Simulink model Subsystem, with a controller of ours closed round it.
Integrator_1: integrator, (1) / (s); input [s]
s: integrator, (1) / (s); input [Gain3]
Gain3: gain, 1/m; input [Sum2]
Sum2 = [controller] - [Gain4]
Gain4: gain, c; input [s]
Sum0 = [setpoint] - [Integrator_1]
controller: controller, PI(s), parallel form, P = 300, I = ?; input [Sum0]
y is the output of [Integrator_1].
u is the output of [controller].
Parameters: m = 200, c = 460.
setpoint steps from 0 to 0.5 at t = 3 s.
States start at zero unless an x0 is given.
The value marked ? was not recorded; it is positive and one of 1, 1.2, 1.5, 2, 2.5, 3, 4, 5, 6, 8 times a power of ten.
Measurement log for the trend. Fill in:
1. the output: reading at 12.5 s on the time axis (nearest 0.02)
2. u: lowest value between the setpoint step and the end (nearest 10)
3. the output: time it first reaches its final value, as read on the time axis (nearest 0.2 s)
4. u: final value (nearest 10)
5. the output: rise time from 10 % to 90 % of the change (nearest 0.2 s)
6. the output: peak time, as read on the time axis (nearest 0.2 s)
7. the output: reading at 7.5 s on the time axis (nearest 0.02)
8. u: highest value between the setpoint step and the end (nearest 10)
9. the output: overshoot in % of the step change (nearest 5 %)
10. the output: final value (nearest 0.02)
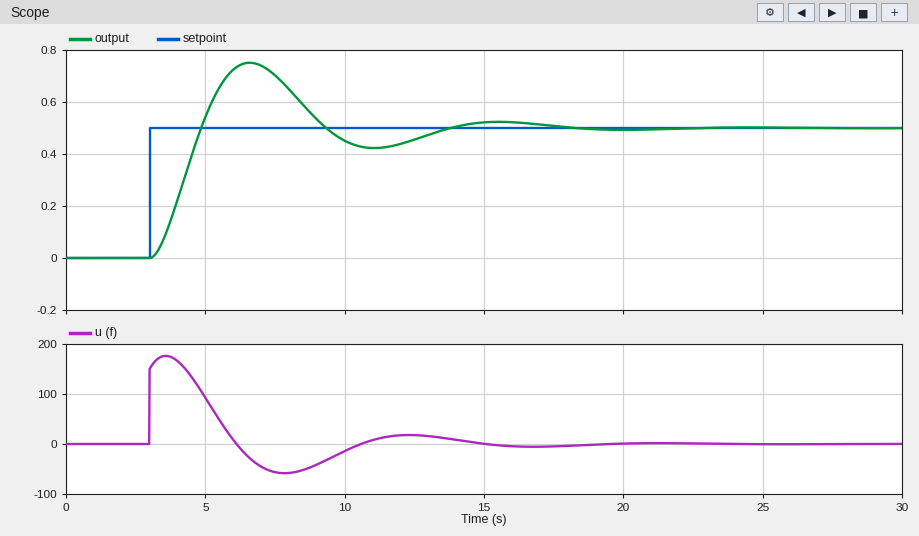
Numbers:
0.46
-60
4.8 s
0
1.2 s
6.6 s
0.70
180
50 %
0.50
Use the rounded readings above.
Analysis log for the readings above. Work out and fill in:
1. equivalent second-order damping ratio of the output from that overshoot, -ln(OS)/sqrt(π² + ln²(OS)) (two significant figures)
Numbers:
0.22
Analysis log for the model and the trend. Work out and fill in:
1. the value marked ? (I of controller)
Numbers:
200
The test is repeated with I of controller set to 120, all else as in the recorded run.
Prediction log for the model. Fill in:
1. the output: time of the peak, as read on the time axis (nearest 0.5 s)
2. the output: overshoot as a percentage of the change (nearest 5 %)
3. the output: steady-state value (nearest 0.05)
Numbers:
7.0 s
35 %
0.50
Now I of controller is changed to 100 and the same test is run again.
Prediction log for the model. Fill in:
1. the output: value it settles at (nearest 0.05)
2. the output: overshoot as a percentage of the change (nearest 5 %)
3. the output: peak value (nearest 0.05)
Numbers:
0.50
30 %
0.65
